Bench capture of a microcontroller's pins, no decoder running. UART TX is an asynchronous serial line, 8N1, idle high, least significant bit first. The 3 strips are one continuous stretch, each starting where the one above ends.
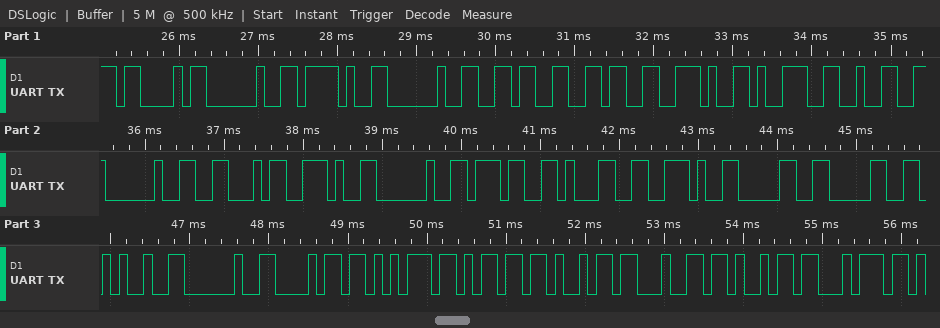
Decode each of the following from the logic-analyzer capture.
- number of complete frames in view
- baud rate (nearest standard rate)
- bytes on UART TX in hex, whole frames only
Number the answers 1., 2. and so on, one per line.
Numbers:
1. 27
2. 9600 baud
3. 43 20 2F 20 36 36 2E 39 32 20 46 2E 20 37 31 2E 30 30 25 20 68 75 6D 69 64 69 74
